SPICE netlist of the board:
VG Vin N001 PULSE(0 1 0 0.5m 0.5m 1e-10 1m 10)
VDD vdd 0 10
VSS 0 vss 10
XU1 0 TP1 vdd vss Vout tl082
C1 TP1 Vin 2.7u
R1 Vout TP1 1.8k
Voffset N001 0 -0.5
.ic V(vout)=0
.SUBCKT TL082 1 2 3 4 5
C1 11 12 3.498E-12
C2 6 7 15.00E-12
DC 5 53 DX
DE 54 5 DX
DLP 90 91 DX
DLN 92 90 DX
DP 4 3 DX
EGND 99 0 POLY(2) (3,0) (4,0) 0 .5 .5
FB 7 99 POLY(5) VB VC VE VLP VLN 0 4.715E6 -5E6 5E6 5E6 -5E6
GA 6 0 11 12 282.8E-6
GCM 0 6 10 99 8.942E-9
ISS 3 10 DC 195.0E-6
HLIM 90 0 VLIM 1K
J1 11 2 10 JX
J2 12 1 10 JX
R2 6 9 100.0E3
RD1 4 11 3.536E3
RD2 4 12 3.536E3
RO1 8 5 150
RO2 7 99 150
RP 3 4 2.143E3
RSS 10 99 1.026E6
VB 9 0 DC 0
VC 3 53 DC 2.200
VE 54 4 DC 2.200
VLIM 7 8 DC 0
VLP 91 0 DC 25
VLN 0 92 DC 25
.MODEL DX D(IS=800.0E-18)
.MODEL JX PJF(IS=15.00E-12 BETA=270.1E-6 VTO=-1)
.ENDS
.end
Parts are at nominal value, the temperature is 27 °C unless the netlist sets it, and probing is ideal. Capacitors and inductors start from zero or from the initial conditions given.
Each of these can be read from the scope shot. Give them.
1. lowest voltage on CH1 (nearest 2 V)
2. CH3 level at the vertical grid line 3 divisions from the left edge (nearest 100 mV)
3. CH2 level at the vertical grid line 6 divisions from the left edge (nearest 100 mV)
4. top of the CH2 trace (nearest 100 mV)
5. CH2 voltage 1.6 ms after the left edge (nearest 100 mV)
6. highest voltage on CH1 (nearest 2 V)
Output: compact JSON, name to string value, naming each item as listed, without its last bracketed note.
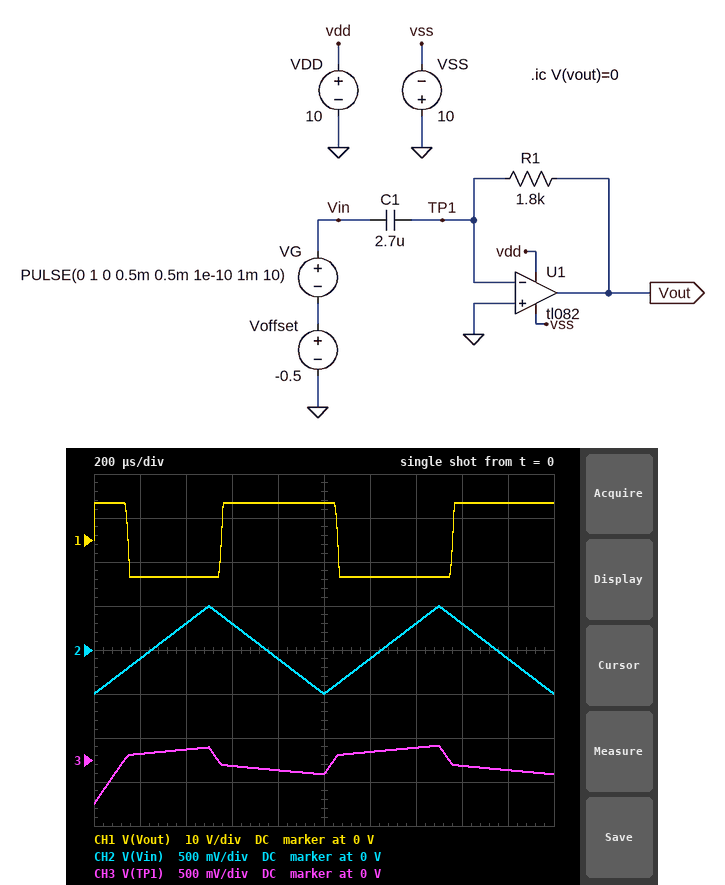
{"lowest voltage on CH1": "-8 V", "CH3 level at the vertical grid line 3 divisions from the left edge": "-100 mV", "CH2 level at the vertical grid line 6 divisions from the left edge": "-100 mV", "top of the CH2 trace": "500 mV", "CH2 voltage 1.6 ms after the left edge": "300 mV", "highest voltage on CH1": "8 V"}
